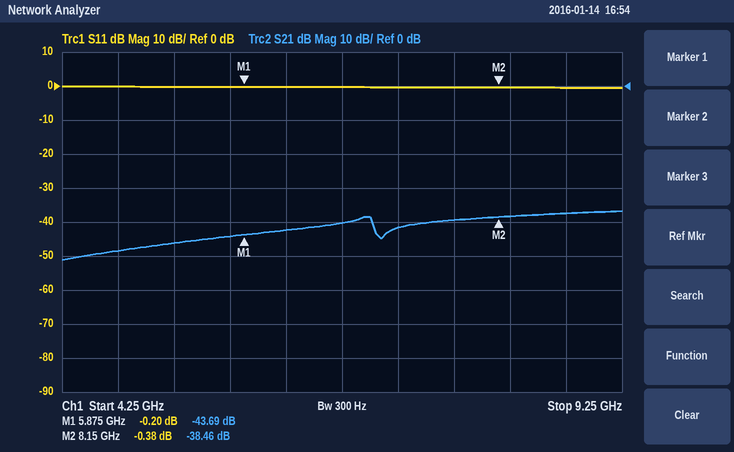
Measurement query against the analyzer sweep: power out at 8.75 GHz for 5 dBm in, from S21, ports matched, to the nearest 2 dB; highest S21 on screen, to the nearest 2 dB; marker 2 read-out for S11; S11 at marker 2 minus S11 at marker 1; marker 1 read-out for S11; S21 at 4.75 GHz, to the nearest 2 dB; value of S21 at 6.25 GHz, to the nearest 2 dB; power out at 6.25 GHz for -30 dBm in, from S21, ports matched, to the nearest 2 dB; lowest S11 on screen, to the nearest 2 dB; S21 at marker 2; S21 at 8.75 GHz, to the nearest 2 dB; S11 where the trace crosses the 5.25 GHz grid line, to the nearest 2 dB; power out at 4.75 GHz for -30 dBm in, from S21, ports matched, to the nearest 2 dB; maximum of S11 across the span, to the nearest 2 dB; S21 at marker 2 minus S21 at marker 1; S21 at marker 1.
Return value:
-32 dBm
-36 dB
-0.38 dB
-0.18 dB
-0.20 dB
-48 dB
-42 dB
-72 dBm
0 dB
-38.46 dB
-38 dB
0 dB
-78 dBm
0 dB
5.23 dB
-43.69 dB
